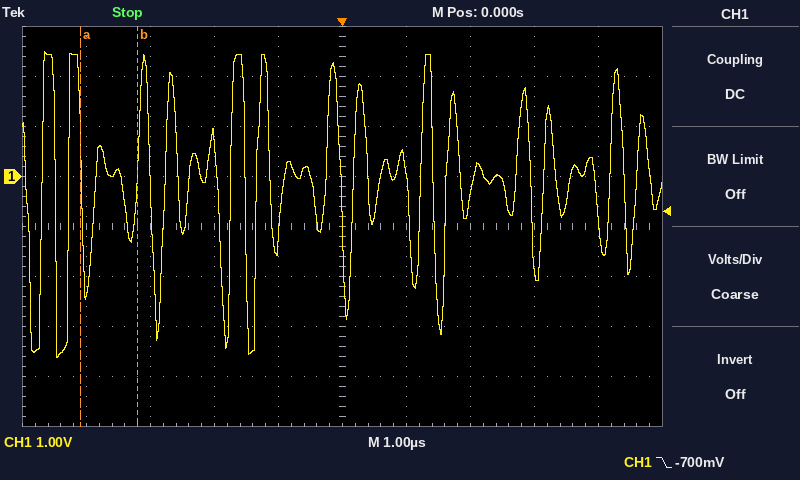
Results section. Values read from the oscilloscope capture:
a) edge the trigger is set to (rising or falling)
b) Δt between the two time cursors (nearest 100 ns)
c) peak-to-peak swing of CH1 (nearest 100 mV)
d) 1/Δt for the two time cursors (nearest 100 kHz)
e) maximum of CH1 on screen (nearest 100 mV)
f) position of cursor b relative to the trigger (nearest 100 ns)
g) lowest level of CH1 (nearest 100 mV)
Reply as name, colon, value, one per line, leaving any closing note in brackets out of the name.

edge the trigger is set to: falling
Δt between the two time cursors: 900 ns
peak-to-peak swing of CH1: 6.1 V
1/Δt for the two time cursors: 1.1 MHz
maximum of CH1 on screen: 2.5 V
position of cursor b relative to the trigger: -3.2 µs
lowest level of CH1: -3.6 V
